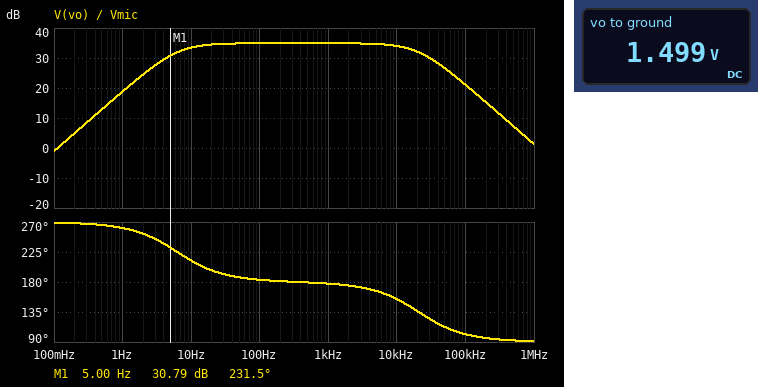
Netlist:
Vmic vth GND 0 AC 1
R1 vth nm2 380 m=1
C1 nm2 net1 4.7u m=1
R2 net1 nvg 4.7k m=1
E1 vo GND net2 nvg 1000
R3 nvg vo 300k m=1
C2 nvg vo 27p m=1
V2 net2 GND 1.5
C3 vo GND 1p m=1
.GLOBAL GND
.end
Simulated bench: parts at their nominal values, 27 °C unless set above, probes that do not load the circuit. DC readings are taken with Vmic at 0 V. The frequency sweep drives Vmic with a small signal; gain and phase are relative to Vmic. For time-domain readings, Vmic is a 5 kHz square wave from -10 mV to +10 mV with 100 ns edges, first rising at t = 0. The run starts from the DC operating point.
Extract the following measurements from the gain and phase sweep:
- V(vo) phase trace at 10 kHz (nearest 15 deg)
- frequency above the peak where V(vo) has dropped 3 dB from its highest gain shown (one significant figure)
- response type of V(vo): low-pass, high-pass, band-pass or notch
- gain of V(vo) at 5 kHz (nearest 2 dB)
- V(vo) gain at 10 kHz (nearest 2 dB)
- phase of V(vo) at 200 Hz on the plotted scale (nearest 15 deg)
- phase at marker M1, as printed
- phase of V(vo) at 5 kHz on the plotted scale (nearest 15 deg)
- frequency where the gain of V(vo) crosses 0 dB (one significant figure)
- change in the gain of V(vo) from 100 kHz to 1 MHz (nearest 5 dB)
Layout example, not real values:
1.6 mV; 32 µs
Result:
150 deg; 20 kHz; band-pass; 34 dB; 34 dB; 180 deg; 231.5 deg; 165 deg; 100 mHz; -20 dB
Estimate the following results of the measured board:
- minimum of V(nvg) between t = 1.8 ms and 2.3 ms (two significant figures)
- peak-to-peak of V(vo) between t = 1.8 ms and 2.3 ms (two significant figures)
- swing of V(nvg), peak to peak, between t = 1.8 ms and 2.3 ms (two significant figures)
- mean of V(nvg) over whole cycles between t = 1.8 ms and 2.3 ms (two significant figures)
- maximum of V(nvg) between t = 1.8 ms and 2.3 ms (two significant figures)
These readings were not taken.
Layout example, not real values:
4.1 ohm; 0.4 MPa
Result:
1.5 V; 1.1 V; 1.1 mV; 1.5 V; 1.5 V
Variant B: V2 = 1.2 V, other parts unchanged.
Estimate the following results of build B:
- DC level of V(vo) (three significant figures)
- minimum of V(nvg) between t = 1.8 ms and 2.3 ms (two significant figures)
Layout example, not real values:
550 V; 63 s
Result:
1.20 V; 1.2 V
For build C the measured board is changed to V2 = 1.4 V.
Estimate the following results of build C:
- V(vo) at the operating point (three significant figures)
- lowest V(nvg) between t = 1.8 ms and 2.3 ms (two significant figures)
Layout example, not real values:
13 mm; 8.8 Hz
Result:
1.40 V; 1.4 V
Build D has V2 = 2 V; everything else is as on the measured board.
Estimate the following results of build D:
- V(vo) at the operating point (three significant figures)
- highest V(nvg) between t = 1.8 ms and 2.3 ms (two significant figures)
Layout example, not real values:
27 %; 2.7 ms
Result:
2.00 V; 2.0 V
